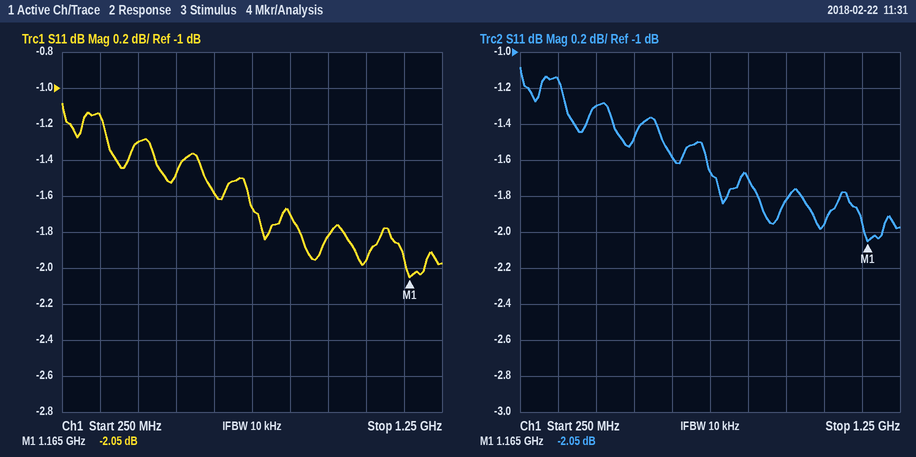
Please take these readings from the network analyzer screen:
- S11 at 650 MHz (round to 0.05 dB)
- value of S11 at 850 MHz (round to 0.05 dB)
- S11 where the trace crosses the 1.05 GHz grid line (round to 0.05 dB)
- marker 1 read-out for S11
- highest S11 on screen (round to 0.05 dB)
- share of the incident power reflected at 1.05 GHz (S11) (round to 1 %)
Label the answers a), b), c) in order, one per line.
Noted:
a) -1.60 dB
b) -1.70 dB
c) -1.95 dB
d) -2.05 dB
e) -1.10 dB
f) 64 %
